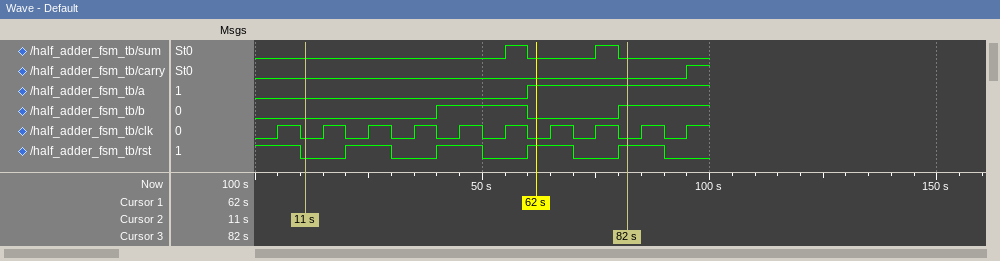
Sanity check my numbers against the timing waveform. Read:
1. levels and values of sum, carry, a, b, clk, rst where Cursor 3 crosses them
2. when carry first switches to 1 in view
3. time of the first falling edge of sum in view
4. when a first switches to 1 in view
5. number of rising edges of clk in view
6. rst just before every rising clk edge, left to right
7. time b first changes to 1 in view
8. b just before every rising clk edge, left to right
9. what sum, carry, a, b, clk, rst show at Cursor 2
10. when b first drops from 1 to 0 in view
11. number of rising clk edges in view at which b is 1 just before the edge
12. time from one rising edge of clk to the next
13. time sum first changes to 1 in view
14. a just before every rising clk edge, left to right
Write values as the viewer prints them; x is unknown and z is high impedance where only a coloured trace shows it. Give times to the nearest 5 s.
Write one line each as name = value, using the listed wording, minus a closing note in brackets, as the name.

levels and values of sum, carry, a, b, clk, rst where Cursor 3 crosses them = sum=0, carry=0, a=1, b=1, clk=0, rst=1
when carry first switches to 1 in view = 95 s
time of the first falling edge of sum in view = 60 s
when a first switches to 1 in view = 60 s
number of rising edges of clk in view = 10
rst just before every rising clk edge, left to right = 1 0 1 0 1 0 1 0 1 0
time b first changes to 1 in view = 40 s
b just before every rising clk edge, left to right = 0 0 0 0 1 1 0 0 1 1
what sum, carry, a, b, clk, rst show at Cursor 2 = sum=0, carry=0, a=0, b=0, clk=0, rst=0
when b first drops from 1 to 0 in view = 60 s
number of rising clk edges in view at which b is 1 just before the edge = 4
time from one rising edge of clk to the next = 10 s
time sum first changes to 1 in view = 55 s
a just before every rising clk edge, left to right = 0 0 0 0 0 0 1 1 1 1
